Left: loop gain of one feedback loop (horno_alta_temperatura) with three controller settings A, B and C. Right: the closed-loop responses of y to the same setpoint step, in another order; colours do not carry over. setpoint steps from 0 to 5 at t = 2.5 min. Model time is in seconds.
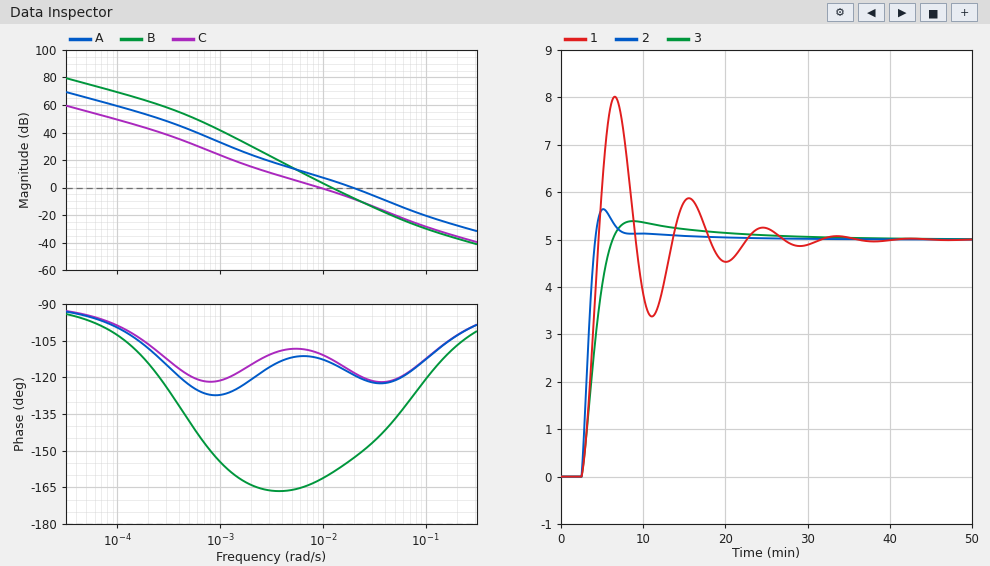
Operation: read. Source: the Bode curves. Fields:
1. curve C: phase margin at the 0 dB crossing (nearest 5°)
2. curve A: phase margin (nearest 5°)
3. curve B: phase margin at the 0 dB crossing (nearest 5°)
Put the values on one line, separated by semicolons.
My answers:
70°; 60°; 20°
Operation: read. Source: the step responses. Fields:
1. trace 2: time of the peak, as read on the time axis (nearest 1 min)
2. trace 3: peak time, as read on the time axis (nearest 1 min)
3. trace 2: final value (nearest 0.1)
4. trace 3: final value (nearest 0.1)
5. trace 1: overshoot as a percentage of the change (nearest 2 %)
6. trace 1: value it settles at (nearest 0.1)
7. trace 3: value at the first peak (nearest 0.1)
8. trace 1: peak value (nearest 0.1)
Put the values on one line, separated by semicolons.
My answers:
5 min; 9 min; 5.0; 5.0; 60 %; 5.0; 5.4; 8.0
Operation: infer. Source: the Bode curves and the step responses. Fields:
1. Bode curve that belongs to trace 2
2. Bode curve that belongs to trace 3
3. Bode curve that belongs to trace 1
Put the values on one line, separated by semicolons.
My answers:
A; C; B
